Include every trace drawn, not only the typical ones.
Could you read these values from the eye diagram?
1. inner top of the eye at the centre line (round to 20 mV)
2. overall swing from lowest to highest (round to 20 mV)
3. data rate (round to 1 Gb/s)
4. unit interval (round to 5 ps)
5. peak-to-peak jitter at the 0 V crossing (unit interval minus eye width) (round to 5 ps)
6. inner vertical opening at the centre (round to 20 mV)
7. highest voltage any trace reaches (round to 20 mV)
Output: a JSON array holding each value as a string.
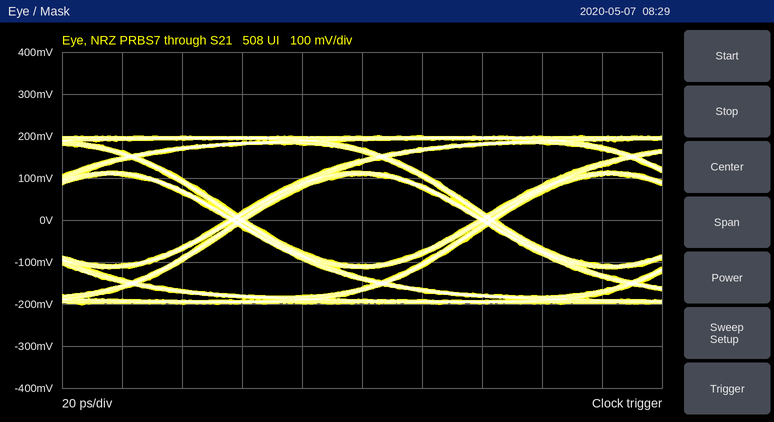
["100 mV", "400 mV", "12 Gb/s", "85 ps", "5 ps", "220 mV", "200 mV"]
